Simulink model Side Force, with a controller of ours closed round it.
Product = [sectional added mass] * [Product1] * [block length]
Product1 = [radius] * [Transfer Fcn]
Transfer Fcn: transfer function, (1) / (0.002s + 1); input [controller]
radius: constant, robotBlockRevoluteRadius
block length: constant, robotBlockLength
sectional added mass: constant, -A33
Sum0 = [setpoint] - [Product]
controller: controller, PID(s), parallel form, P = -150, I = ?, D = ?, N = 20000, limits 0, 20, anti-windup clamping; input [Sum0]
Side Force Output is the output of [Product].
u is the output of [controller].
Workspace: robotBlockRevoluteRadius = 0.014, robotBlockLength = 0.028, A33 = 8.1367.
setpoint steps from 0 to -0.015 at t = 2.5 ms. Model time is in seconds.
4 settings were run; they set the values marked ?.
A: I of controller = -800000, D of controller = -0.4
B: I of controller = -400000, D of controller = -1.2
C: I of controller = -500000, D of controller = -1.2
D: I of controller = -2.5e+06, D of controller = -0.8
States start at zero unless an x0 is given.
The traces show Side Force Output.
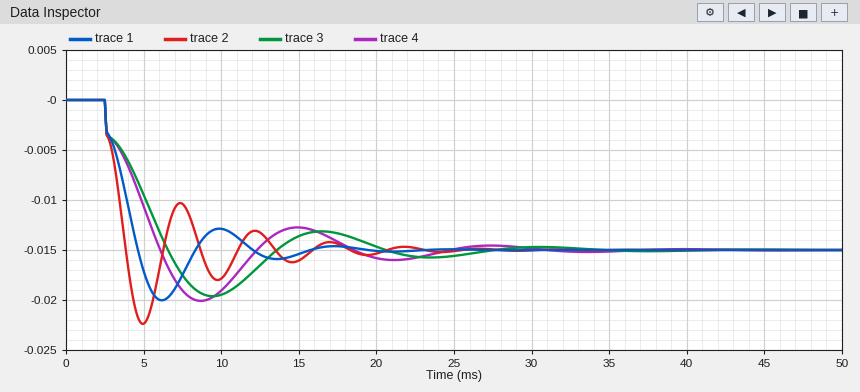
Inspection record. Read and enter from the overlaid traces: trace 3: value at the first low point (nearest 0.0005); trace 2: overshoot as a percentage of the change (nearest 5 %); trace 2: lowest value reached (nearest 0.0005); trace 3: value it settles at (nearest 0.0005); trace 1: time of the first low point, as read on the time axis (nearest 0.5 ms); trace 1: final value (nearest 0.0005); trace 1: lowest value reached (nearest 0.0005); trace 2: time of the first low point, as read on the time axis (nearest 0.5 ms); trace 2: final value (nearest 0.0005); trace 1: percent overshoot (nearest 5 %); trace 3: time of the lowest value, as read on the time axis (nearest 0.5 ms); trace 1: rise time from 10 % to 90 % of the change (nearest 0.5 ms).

-0.0195
50 %
-0.0225
-0.0150
6.0 ms
-0.0150
-0.0200
5.0 ms
-0.0150
35 %
9.5 ms
2.0 ms
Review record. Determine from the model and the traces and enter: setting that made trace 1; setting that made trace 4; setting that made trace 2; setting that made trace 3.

A
C
D
B
